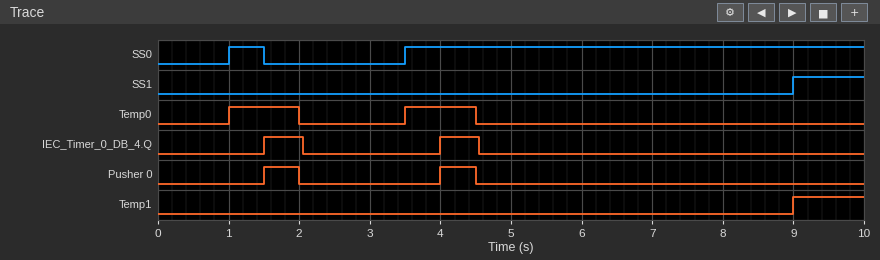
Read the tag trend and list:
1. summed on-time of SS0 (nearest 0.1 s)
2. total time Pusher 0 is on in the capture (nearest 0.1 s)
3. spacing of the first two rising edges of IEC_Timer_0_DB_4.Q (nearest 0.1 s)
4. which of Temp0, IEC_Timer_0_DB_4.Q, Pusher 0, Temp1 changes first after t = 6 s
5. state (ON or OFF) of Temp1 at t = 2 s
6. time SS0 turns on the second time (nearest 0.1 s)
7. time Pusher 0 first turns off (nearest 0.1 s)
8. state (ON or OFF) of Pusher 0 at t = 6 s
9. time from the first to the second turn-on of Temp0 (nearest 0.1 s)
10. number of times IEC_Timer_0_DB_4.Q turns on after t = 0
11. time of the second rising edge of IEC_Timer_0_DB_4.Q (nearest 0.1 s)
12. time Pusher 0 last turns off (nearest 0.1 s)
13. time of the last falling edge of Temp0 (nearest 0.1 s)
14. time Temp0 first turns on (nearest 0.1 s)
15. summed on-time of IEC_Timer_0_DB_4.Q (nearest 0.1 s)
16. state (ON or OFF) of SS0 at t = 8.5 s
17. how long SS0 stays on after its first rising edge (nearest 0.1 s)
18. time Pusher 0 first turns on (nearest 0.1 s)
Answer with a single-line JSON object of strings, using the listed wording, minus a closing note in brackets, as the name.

{"summed on-time of SS0": "7.0 s", "total time Pusher 0 is on in the capture": "1.0 s", "spacing of the first two rising edges of IEC_Timer_0_DB_4.Q": "2.5 s", "which of Temp0, IEC_Timer_0_DB_4.Q, Pusher 0, Temp1 changes first after t = 6 s": "Temp1", "state (ON or OFF) of Temp1 at t = 2 s": "OFF", "time SS0 turns on the second time": "3.5 s", "time Pusher 0 first turns off": "2.0 s", "state (ON or OFF) of Pusher 0 at t = 6 s": "OFF", "time from the first to the second turn-on of Temp0": "2.5 s", "number of times IEC_Timer_0_DB_4.Q turns on after t = 0": "2", "time of the second rising edge of IEC_Timer_0_DB_4.Q": "4.0 s", "time Pusher 0 last turns off": "4.5 s", "time of the last falling edge of Temp0": "4.5 s", "time Temp0 first turns on": "1.0 s", "summed on-time of IEC_Timer_0_DB_4.Q": "1.1 s", "state (ON or OFF) of SS0 at t = 8.5 s": "ON", "how long SS0 stays on after its first rising edge": "0.5 s", "time Pusher 0 first turns on": "1.5 s"}
